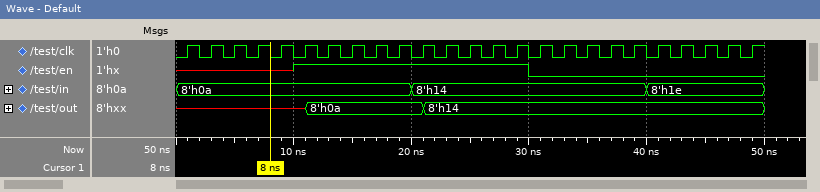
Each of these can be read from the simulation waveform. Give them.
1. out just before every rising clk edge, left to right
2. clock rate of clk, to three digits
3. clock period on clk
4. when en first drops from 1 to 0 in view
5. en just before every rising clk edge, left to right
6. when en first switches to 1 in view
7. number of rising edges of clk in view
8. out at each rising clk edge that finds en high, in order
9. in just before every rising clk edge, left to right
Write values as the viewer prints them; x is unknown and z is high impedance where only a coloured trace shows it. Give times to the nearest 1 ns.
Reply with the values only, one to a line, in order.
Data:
x, x, x, x, x, x, 8'h0a, 8'h0a, 8'h0a, 8'h0a, 8'h0a, 8'h14, 8'h14, 8'h14, 8'h14, 8'h14, 8'h14, 8'h14, 8'h14, 8'h14, 8'h14, 8'h14, 8'h14, 8'h14, 8'h14
500 MHz
2 ns
30 ns
x x x x x 1 1 1 1 1 1 1 1 1 1 0 0 0 0 0 0 0 0 0 0
10 ns
25
x, 8'h0a, 8'h0a, 8'h0a, 8'h0a, 8'h0a, 8'h14, 8'h14, 8'h14, 8'h14
8'h0a, 8'h0a, 8'h0a, 8'h0a, 8'h0a, 8'h0a, 8'h0a, 8'h0a, 8'h0a, 8'h0a, 8'h14, 8'h14, 8'h14, 8'h14, 8'h14, 8'h14, 8'h14, 8'h14, 8'h14, 8'h14, 8'h1e, 8'h1e, 8'h1e, 8'h1e, 8'h1e
